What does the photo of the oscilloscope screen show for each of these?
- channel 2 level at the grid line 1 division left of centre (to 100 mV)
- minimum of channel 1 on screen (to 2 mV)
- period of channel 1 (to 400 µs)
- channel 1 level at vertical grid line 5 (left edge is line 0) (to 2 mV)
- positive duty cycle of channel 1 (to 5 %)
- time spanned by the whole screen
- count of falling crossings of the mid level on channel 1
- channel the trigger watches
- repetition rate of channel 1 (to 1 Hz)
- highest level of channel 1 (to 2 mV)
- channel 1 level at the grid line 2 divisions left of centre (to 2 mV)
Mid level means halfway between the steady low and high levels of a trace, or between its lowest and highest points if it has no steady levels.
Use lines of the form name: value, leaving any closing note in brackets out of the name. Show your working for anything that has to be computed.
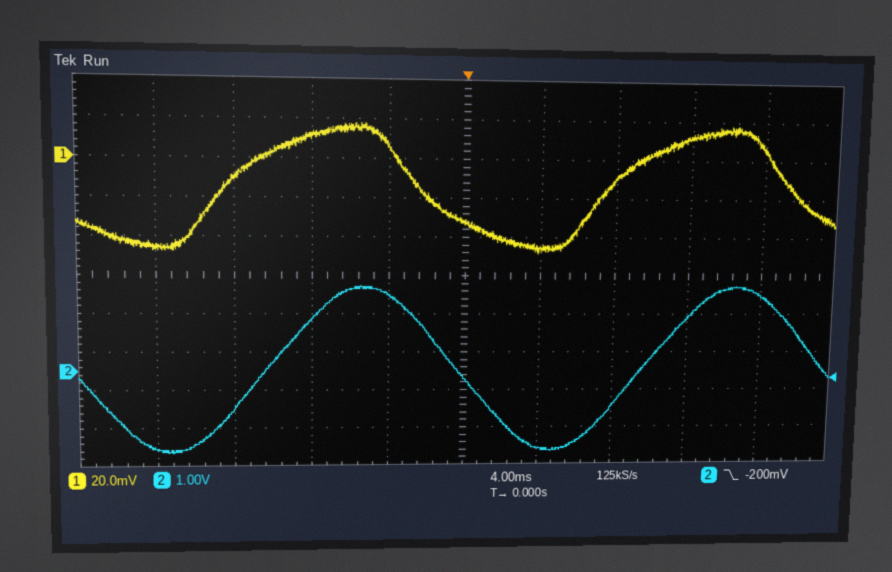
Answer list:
channel 2 level at the grid line 1 division left of centre: 2.0 V
minimum of channel 1 on screen: -48 mV
period of channel 1: 20.0 ms
channel 1 level at vertical grid line 5 (left edge is line 0): -32 mV
positive duty cycle of channel 1: 50 %
time spanned by the whole screen: 40 ms
count of falling crossings of the mid level on channel 1: 2
channel the trigger watches: channel 2
repetition rate of channel 1: 1 / 20.0 ms ≈ 50 Hz
highest level of channel 1: 18 mV
channel 1 level at the grid line 2 divisions left of centre: 12 mV
